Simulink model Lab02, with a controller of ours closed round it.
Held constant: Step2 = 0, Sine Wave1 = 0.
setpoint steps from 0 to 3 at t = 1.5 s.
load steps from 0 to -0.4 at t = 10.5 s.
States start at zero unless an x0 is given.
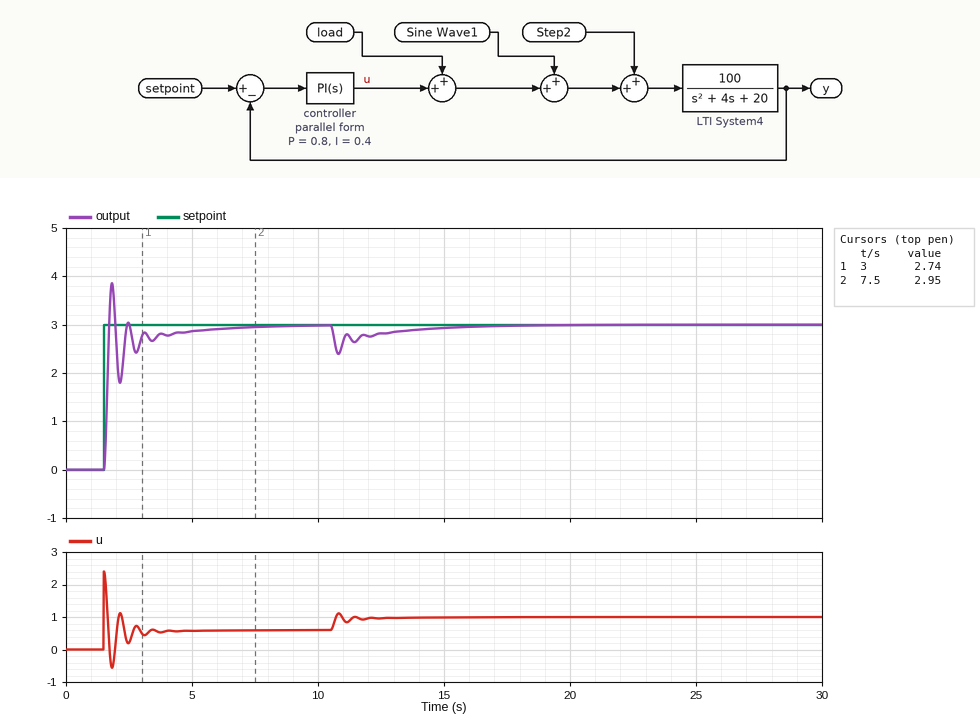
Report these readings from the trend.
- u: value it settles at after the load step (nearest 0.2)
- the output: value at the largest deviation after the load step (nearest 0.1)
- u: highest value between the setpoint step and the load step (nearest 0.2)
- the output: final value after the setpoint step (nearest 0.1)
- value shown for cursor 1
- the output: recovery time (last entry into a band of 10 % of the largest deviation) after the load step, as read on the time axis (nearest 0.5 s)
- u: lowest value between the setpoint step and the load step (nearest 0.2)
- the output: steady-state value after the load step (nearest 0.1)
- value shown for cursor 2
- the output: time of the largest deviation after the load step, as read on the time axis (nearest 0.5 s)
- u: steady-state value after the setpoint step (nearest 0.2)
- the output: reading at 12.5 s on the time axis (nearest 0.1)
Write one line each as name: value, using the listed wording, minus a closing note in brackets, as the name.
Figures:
u: value it settles at after the load step: 1.0
the output: value at the largest deviation after the load step: 2.4
u: highest value between the setpoint step and the load step: 2.4
the output: final value after the setpoint step: 3.0
value shown for cursor 1: 2.74
the output: recovery time (last entry into a band of 10 % of the largest deviation) after the load step, as read on the time axis: 15.5 s
u: lowest value between the setpoint step and the load step: -0.6
the output: steady-state value after the load step: 3.0
value shown for cursor 2: 2.95
the output: time of the largest deviation after the load step, as read on the time axis: 11.0 s
u: steady-state value after the setpoint step: 0.6
the output: reading at 12.5 s on the time axis: 2.8
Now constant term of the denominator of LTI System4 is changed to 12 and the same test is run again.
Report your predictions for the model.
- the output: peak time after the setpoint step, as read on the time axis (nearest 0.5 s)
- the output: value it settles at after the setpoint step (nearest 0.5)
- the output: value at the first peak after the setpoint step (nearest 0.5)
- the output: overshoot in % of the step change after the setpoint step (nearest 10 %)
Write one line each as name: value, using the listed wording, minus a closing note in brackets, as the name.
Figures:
the output: peak time after the setpoint step, as read on the time axis: 2.0 s
the output: value it settles at after the setpoint step: 3.0
the output: value at the first peak after the setpoint step: 4.0
the output: overshoot in % of the step change after the setpoint step: 40 %
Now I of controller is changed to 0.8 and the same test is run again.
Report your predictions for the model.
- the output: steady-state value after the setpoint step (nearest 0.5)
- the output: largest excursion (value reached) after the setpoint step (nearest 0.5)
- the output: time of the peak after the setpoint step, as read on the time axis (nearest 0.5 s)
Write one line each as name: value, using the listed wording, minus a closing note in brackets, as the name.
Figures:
the output: steady-state value after the setpoint step: 3.0
the output: largest excursion (value reached) after the setpoint step: 4.0
the output: time of the peak after the setpoint step, as read on the time axis: 2.0 s
